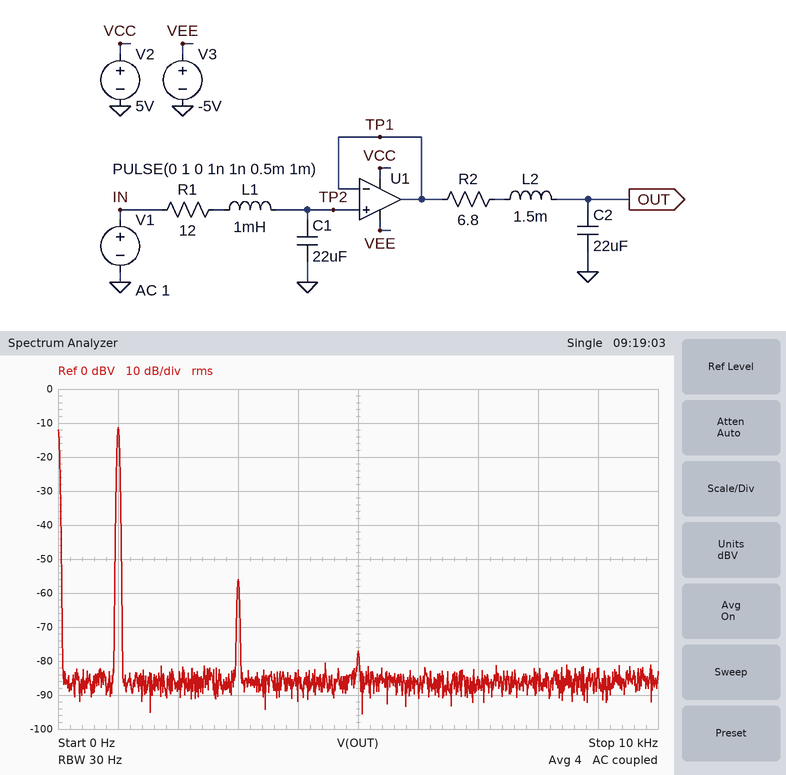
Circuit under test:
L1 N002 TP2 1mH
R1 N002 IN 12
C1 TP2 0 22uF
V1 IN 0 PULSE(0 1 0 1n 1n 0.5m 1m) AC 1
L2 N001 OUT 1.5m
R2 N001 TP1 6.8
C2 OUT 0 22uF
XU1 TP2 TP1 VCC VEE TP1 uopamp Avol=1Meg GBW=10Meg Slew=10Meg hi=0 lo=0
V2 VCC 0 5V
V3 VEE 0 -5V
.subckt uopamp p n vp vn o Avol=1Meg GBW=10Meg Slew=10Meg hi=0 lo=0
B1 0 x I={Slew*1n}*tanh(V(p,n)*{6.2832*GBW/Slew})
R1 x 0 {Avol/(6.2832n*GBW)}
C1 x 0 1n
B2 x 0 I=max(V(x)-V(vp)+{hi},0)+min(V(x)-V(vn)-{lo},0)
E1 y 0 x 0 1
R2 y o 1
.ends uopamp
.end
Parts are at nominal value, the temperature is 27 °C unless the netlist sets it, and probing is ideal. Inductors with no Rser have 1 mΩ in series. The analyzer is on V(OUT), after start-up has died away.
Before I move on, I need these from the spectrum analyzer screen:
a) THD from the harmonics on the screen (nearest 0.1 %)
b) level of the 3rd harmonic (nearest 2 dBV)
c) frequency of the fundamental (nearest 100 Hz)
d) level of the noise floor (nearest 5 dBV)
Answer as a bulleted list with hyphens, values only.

- 0.6 %
- -56 dBV
- 1.0 kHz
- -85 dBV
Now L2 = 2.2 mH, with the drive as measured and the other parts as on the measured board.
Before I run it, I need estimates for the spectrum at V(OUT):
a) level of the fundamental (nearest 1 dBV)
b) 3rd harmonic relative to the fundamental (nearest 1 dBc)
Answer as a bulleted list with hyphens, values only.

- -14 dBV
- -46 dBc
